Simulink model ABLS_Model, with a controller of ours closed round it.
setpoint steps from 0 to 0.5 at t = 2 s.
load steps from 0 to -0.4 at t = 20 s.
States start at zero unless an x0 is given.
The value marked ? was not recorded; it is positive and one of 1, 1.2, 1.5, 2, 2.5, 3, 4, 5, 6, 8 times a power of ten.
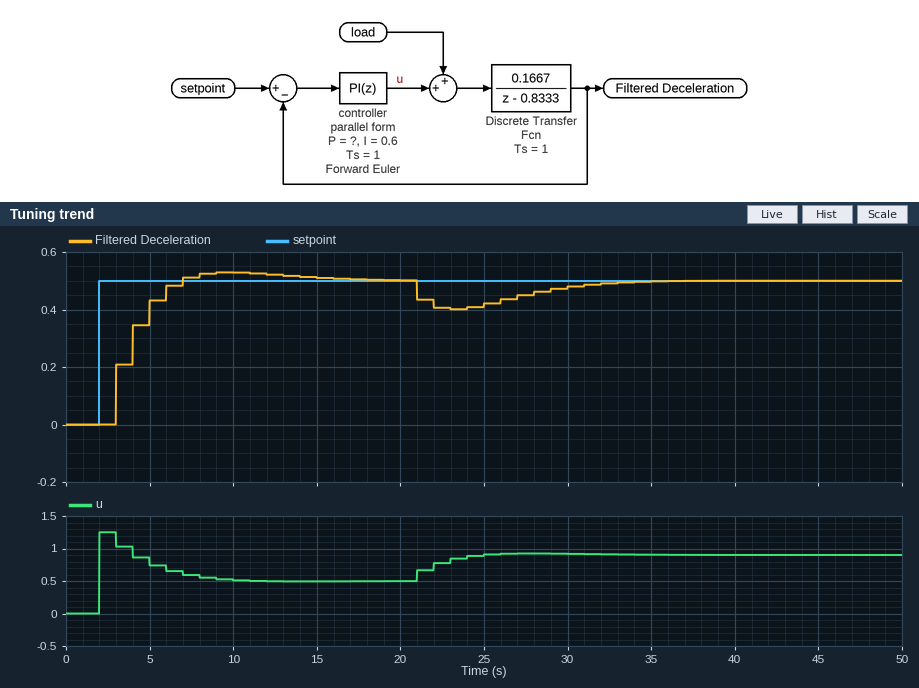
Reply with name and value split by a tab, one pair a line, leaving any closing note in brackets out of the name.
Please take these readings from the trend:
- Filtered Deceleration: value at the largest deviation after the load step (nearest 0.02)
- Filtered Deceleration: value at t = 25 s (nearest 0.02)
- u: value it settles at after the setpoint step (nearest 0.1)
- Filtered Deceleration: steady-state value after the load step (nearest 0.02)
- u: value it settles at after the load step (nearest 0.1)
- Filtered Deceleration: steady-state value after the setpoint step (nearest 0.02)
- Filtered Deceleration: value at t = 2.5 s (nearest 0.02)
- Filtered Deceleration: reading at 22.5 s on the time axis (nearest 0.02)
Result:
Filtered Deceleration: value at the largest deviation after the load step	0.40
Filtered Deceleration: value at t = 25 s	0.42
u: value it settles at after the setpoint step	0.5
Filtered Deceleration: steady-state value after the load step	0.50
u: value it settles at after the load step	0.9
Filtered Deceleration: steady-state value after the setpoint step	0.50
Filtered Deceleration: value at t = 2.5 s	0.00
Filtered Deceleration: reading at 22.5 s on the time axis	0.40
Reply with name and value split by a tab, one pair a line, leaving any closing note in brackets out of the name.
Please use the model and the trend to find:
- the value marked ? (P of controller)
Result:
the value marked ?	2.5
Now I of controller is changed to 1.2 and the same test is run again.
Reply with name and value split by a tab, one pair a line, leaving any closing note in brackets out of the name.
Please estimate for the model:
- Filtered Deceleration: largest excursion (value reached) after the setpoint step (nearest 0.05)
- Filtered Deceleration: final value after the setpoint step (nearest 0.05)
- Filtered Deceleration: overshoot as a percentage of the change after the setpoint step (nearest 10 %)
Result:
Filtered Deceleration: largest excursion (value reached) after the setpoint step	0.65
Filtered Deceleration: final value after the setpoint step	0.50
Filtered Deceleration: overshoot as a percentage of the change after the setpoint step	30 %
